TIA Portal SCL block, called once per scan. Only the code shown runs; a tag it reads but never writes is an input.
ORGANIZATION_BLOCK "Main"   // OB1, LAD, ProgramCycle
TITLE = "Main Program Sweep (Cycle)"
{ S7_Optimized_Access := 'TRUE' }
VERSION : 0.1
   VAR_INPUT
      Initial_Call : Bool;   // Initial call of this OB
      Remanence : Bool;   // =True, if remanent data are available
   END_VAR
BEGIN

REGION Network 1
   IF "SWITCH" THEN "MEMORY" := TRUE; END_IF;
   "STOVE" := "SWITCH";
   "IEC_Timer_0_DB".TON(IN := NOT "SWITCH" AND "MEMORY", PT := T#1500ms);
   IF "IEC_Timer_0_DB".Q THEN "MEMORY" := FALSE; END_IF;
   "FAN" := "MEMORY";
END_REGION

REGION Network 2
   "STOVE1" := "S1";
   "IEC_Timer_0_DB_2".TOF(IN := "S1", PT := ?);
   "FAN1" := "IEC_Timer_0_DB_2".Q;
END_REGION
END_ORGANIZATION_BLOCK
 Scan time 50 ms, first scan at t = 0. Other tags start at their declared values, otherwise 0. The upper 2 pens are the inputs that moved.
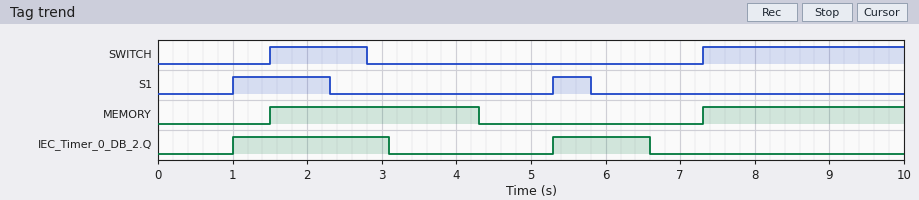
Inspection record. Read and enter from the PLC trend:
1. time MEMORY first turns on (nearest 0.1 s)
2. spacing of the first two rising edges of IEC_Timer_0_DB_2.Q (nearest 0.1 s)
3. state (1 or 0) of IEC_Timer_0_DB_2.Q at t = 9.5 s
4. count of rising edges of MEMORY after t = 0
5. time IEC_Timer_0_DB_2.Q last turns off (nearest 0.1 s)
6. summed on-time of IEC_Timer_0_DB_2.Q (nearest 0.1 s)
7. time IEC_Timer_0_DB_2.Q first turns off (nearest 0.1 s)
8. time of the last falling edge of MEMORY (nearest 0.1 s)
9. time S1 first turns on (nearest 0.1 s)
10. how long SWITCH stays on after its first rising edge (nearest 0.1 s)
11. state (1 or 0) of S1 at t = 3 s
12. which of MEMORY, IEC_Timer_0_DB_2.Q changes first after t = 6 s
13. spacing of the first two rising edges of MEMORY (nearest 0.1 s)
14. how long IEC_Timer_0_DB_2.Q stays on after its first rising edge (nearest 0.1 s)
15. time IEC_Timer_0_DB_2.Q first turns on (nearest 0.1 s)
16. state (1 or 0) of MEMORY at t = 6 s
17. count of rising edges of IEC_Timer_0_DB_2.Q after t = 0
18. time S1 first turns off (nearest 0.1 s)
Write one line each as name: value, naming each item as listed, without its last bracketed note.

time MEMORY first turns on: 1.5 s
spacing of the first two rising edges of IEC_Timer_0_DB_2.Q: 4.3 s
state (1 or 0) of IEC_Timer_0_DB_2.Q at t = 9.5 s: 0
count of rising edges of MEMORY after t = 0: 2
time IEC_Timer_0_DB_2.Q last turns off: 6.6 s
summed on-time of IEC_Timer_0_DB_2.Q: 3.4 s
time IEC_Timer_0_DB_2.Q first turns off: 3.1 s
time of the last falling edge of MEMORY: 4.3 s
time S1 first turns on: 1.0 s
how long SWITCH stays on after its first rising edge: 1.3 s
state (1 or 0) of S1 at t = 3 s: 0
which of MEMORY, IEC_Timer_0_DB_2.Q changes first after t = 6 s: IEC_Timer_0_DB_2.Q
spacing of the first two rising edges of MEMORY: 5.8 s
how long IEC_Timer_0_DB_2.Q stays on after its first rising edge: 2.1 s
time IEC_Timer_0_DB_2.Q first turns on: 1.0 s
state (1 or 0) of MEMORY at t = 6 s: 0
count of rising edges of IEC_Timer_0_DB_2.Q after t = 0: 2
time S1 first turns off: 2.3 s
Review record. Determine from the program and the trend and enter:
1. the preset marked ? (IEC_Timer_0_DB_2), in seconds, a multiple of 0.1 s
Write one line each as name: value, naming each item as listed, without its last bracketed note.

the preset marked ? (IEC_Timer_0_DB_2), in seconds, a multiple of 0.1 s: 0.8 s
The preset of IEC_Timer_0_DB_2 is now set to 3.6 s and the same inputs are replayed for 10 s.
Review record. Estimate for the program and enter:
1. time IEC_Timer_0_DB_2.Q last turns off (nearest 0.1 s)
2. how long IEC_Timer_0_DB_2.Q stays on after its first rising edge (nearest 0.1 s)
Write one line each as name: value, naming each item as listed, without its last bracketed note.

time IEC_Timer_0_DB_2.Q last turns off: 9.4 s
how long IEC_Timer_0_DB_2.Q stays on after its first rising edge: 8.4 s
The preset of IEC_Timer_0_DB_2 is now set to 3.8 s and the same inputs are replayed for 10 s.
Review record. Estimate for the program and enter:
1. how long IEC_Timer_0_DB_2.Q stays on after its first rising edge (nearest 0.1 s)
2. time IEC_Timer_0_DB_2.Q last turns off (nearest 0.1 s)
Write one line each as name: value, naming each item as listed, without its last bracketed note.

how long IEC_Timer_0_DB_2.Q stays on after its first rising edge: 8.6 s
time IEC_Timer_0_DB_2.Q last turns off: 9.6 s
